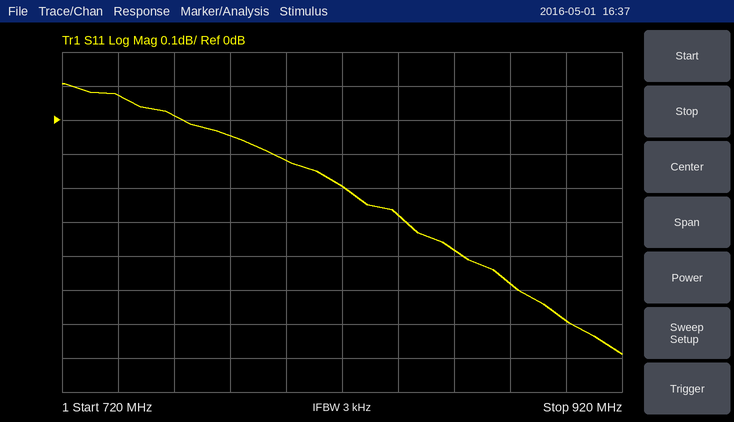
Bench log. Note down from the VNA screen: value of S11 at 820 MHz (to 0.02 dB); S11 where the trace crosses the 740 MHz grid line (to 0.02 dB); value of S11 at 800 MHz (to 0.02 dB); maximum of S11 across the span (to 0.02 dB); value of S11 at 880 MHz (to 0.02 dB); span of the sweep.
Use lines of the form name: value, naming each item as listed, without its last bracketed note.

value of S11 at 820 MHz: -0.20 dB
S11 where the trace crosses the 740 MHz grid line: 0.08 dB
value of S11 at 800 MHz: -0.12 dB
maximum of S11 across the span: 0.10 dB
value of S11 at 880 MHz: -0.48 dB
span of the sweep: 200 MHz
